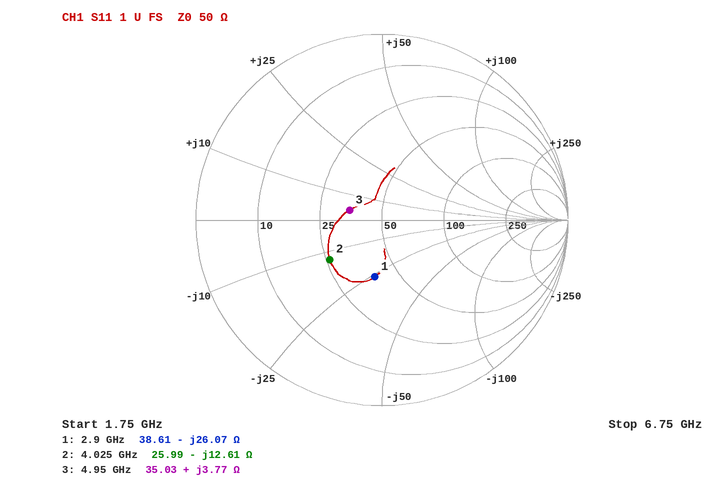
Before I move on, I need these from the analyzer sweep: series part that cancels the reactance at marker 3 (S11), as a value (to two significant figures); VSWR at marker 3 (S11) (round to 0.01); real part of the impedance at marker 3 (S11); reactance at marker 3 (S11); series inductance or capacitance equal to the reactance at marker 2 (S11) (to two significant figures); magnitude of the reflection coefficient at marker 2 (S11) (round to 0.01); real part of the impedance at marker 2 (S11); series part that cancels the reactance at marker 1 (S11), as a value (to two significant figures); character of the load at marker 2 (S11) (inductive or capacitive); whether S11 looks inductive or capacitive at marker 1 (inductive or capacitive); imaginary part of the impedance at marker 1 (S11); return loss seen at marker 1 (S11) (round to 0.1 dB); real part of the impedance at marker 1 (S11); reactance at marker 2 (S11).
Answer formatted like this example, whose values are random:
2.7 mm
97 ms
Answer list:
8.5 pF
1.44
35.03 Ω
+3.77 Ω
3.1 pF
0.35
25.99 Ω
1.4 nH
capacitive
capacitive
-26.07 Ω
10.2 dB
38.61 Ω
-12.61 Ω
